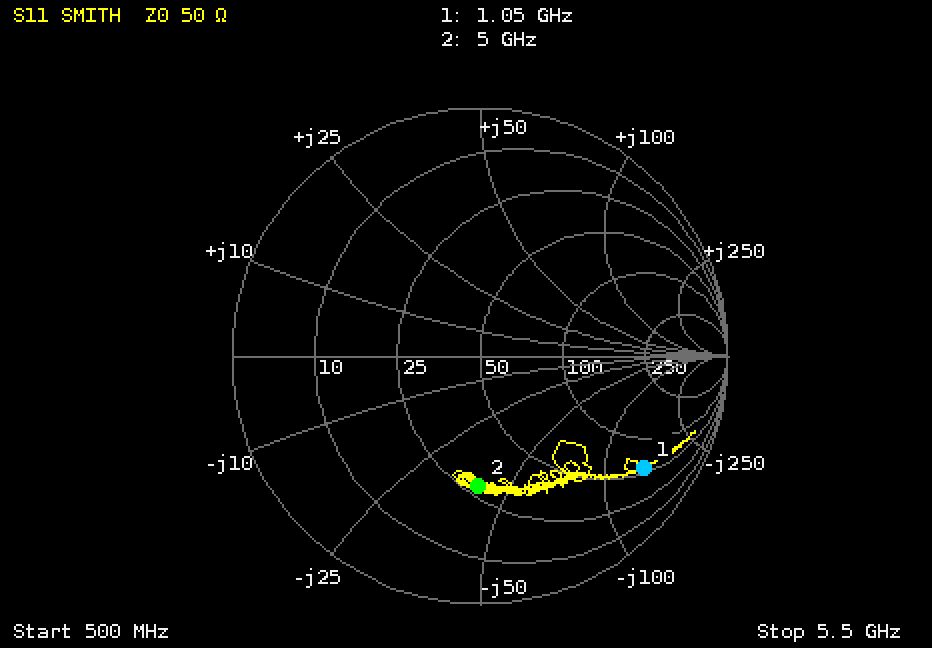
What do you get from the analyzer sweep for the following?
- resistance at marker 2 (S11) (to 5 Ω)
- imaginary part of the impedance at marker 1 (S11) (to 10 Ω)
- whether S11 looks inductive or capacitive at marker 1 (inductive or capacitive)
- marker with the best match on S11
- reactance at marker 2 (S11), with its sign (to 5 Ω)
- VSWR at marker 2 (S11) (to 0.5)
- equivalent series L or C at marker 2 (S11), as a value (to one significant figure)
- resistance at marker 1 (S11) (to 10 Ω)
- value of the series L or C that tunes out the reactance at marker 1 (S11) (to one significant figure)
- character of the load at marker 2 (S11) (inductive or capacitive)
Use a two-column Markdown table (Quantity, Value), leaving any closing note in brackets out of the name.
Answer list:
| Quantity | Value |
|---|---|
| resistance at marker 2 (S11) | 30 Ω |
| imaginary part of the impedance at marker 1 (S11) | -140 Ω |
| whether S11 looks inductive or capacitive at marker 1 | capacitive |
| marker with the best match on S11 | marker 2 |
| reactance at marker 2 (S11), with its sign | -40 Ω |
| VSWR at marker 2 (S11) | 3.0 |
| equivalent series L or C at marker 2 (S11), as a value | 800 fF |
| resistance at marker 1 (S11) | 60 Ω |
| value of the series L or C that tunes out the reactance at marker 1 (S11) | 20 nH |
| character of the load at marker 2 (S11) | capacitive |
